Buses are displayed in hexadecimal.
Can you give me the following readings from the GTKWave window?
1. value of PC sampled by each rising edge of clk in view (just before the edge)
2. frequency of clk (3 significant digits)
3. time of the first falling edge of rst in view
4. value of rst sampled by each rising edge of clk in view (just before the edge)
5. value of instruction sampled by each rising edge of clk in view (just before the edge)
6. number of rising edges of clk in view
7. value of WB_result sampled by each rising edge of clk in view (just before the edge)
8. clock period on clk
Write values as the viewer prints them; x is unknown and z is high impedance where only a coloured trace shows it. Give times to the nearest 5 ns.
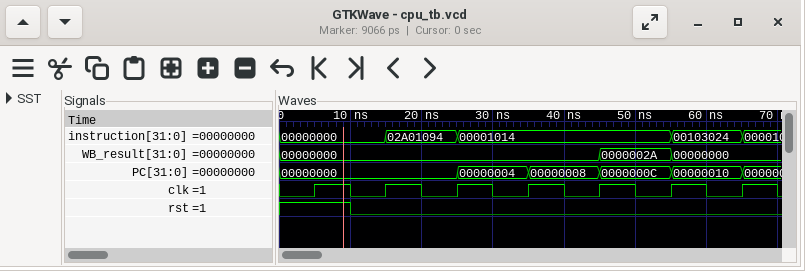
00000000, 00000000, 00000000, 00000004, 00000008, 0000000C, 00000010
100 MHz
10 ns
1 0 0 0 0 0 0
00000000, 00000000, 02A01094, 00001014, 00001014, 00001014, 00103024
7
00000000, 00000000, 00000000, 00000000, 00000000, 0000002A, 00000000
10 ns
